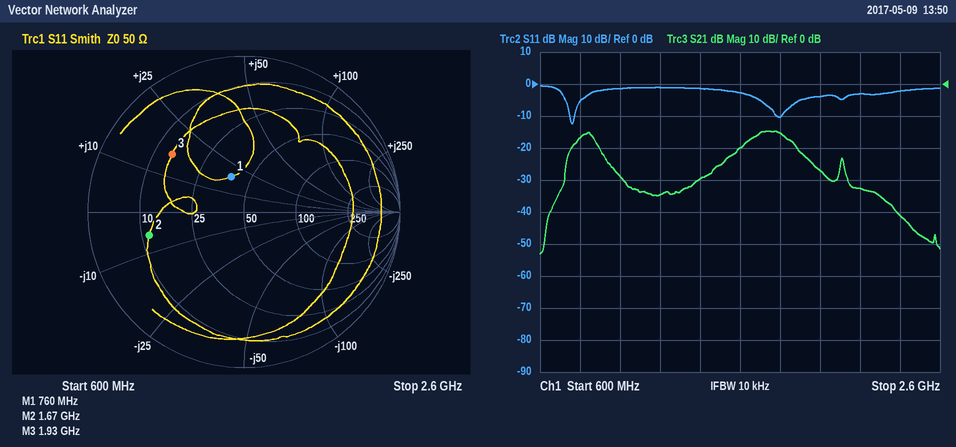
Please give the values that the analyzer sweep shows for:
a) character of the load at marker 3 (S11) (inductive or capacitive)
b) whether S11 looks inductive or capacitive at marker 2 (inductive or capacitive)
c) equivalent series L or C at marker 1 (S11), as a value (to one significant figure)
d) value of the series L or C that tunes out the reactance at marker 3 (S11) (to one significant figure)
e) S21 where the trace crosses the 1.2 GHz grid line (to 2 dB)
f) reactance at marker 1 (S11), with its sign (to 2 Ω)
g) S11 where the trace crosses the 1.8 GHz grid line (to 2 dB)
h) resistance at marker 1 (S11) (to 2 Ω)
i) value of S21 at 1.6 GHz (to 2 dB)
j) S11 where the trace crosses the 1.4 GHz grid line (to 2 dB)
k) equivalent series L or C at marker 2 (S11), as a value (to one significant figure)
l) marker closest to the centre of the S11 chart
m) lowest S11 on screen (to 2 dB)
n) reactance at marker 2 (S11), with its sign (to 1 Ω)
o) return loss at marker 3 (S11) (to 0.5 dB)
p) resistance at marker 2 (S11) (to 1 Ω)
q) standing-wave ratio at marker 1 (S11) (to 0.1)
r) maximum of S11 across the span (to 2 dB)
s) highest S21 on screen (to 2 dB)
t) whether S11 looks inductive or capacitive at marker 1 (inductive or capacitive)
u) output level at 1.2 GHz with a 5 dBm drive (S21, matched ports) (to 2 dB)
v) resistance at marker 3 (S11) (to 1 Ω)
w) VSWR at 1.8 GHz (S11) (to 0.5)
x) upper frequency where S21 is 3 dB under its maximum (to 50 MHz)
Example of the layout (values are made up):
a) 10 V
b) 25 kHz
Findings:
a) inductive
b) capacitive
c) 4 nH
d) 5 pF
e) -34 dB
f) +18 Ω
g) -10 dB
h) 38 Ω
i) -20 dB
j) -2 dB
k) 20 pF
l) marker 1
m) -12 dB
n) -6 Ω
o) 4.5 dB
p) 12 Ω
q) 1.6
r) 0 dB
s) -14 dB
t) inductive
u) -30 dBm
v) 14 Ω
w) 2.0
x) 1.85 GHz
